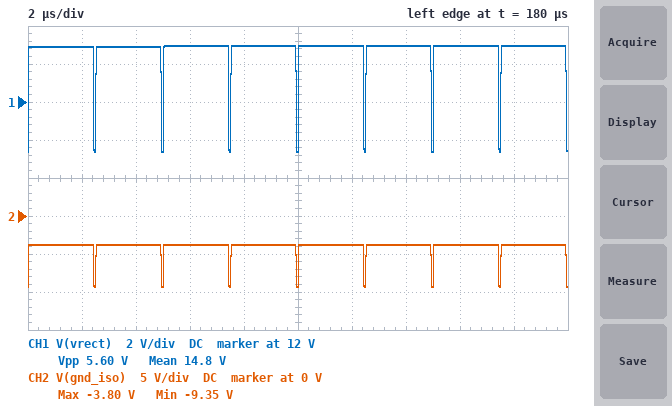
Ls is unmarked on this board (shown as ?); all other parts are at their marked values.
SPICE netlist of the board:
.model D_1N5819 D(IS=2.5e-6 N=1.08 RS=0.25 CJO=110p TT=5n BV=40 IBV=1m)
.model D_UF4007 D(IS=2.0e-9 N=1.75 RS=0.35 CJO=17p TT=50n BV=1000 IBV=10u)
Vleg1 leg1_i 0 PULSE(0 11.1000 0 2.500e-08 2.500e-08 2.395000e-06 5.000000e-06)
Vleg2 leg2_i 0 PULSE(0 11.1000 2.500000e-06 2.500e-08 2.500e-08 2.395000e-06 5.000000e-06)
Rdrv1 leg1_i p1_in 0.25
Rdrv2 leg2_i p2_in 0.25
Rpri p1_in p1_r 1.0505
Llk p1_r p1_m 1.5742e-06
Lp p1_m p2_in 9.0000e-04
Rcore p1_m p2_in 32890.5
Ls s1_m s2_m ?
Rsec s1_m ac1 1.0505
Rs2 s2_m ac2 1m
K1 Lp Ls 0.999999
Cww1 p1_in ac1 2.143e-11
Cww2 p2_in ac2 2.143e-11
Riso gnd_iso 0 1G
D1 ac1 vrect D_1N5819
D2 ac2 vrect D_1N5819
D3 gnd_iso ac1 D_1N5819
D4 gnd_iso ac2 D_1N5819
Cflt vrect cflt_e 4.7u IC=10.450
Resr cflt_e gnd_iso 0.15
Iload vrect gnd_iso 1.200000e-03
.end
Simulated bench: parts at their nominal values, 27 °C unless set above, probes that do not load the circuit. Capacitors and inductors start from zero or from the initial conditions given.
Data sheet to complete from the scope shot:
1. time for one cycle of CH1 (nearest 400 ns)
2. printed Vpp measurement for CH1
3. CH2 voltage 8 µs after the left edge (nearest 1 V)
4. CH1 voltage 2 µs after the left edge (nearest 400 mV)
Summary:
2.4 µs
5.60 V
-4 V
14.8 V
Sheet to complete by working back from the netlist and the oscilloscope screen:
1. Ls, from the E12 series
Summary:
2.7 mH
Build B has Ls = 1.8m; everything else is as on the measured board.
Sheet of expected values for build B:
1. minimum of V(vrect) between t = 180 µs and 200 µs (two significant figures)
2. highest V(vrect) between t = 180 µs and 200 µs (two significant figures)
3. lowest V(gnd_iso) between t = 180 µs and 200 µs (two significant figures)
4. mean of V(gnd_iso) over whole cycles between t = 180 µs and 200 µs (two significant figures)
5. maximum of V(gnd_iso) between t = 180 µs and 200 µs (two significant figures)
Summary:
7.7 V
13 V
-7.7 V
-2.3 V
-2.1 V
